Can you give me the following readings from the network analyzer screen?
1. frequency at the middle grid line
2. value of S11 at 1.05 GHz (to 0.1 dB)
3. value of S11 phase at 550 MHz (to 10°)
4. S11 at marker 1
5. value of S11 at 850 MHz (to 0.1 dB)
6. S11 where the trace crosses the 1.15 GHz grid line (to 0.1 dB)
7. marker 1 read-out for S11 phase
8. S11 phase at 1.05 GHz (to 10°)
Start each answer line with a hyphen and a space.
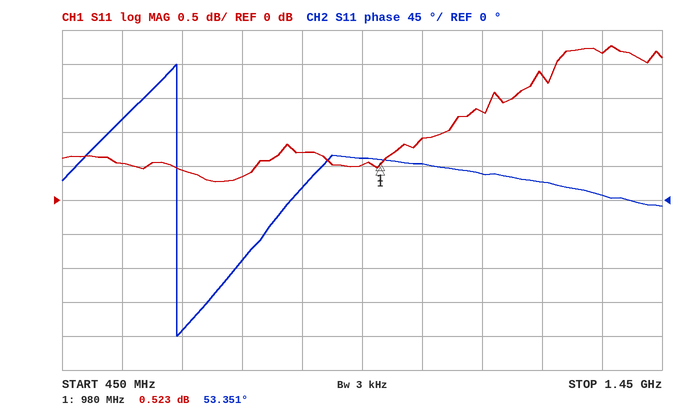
- 950 MHz
- 0.9 dB
- 110°
- 0.523 dB
- 0.7 dB
- 1.3 dB
- 53.351°
- 50°
